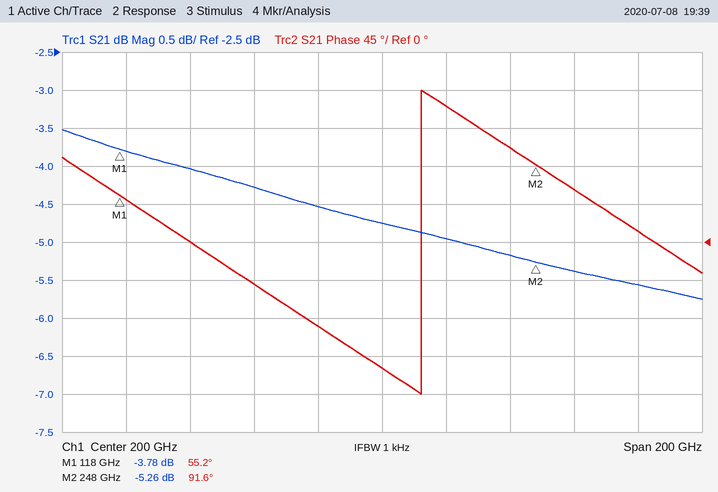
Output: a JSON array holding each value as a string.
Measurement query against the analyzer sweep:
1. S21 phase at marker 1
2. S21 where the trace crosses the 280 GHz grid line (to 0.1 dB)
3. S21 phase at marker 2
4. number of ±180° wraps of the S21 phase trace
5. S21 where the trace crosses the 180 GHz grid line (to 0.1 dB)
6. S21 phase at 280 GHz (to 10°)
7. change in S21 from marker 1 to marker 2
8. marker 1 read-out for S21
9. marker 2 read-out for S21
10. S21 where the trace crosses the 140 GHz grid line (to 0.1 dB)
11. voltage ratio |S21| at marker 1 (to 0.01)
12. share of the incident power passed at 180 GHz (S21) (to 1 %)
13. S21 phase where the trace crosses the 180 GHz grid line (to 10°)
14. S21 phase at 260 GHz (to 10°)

["55.2°", "-5.6 dB", "91.6°", "1", "-4.5 dB", "10°", "-1.48 dB", "-3.78 dB", "-5.26 dB", "-4.0 dB", "0.65", "35 %", "-100°", "60°"]
